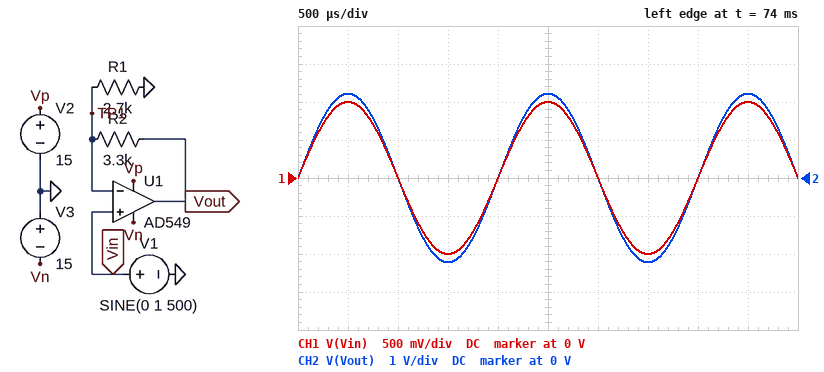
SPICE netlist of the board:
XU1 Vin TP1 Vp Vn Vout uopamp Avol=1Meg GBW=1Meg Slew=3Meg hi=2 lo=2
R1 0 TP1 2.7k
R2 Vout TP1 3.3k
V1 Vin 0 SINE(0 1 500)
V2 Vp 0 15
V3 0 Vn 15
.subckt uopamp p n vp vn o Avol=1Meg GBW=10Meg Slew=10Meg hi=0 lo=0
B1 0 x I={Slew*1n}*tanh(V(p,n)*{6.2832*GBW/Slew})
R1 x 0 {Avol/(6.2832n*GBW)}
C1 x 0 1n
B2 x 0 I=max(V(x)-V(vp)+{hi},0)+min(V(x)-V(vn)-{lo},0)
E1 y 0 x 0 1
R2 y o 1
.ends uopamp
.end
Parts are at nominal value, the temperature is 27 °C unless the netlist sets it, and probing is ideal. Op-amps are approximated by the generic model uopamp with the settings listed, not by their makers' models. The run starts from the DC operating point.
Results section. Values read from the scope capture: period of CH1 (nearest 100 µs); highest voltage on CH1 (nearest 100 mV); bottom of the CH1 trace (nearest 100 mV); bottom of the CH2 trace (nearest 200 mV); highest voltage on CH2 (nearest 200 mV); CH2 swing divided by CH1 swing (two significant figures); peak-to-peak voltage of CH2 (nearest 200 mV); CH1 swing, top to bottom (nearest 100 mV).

2.0 ms
1.0 V
-1.0 V
-2.2 V
2.2 V
2.2
4.4 V
2.0 V
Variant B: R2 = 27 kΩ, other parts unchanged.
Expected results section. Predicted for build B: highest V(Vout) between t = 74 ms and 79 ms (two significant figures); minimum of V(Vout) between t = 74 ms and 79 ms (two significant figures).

11 V
-11 V
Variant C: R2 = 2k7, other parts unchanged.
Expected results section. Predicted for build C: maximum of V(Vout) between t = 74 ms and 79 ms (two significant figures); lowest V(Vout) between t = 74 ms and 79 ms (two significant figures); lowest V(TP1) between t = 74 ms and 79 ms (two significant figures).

2.0 V
-2.0 V
-1.0 V
